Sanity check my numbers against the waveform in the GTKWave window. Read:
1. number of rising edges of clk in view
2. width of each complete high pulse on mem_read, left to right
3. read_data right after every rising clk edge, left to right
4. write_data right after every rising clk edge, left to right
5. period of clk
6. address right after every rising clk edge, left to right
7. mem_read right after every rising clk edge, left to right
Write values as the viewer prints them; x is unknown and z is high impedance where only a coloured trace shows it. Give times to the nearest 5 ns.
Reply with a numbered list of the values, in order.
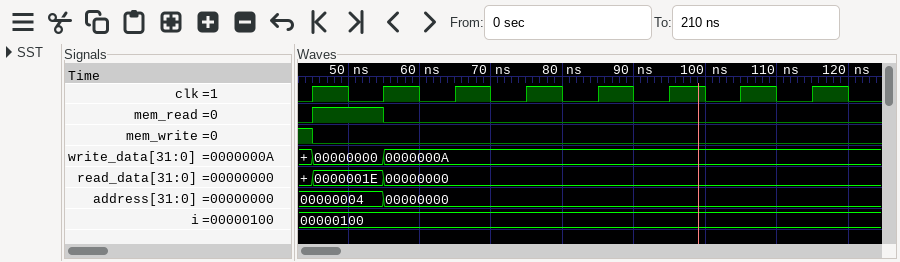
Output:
1. 8
2. 10 ns
3. 0000001E, 00000000, 00000000, 00000000, 00000000, 00000000, 00000000, 00000000
4. 00000000, 0000000A, 0000000A, 0000000A, 0000000A, 0000000A, 0000000A, 0000000A
5. 10 ns
6. 00000004, 00000000, 00000000, 00000000, 00000000, 00000000, 00000000, 00000000
7. 1 0 0 0 0 0 0 0
